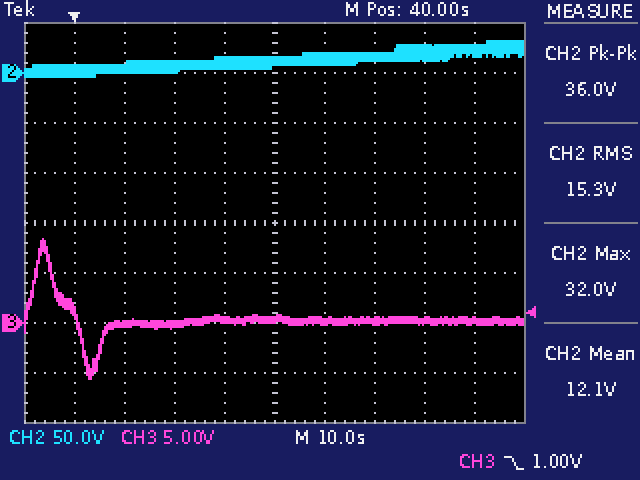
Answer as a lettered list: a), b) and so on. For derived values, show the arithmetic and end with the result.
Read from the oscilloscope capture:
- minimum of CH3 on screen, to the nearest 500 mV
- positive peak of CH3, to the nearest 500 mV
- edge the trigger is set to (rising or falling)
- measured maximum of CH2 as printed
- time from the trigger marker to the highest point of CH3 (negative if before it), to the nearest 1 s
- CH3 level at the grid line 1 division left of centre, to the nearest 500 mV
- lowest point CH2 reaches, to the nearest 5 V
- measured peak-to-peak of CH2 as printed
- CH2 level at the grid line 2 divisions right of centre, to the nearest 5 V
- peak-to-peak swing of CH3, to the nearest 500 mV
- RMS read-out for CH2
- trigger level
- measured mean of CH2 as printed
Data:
a) -5.5 V
b) 8.5 V
c) falling
d) 32.0 V
e) -6 s
f) 500 mV
g) -5 V
h) 36.0 V
i) 15 V
j) 8.5 V − (-5.5 V) = 14.0 V
k) 15.3 V
l) 1.00 V
m) 12.1 V
